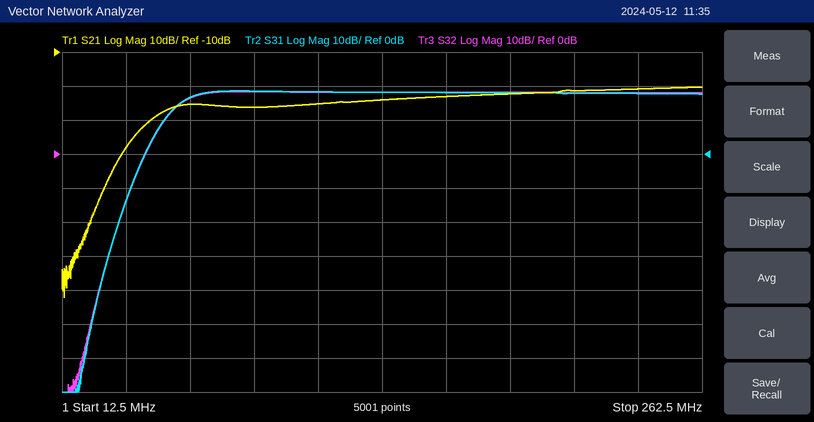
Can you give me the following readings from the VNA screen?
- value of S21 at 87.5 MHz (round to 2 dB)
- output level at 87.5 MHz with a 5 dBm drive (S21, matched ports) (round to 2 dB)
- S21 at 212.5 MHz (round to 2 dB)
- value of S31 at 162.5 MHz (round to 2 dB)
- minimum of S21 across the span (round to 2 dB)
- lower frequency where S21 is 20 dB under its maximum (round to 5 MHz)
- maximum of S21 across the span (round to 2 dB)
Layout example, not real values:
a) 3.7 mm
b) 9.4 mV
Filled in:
a) -26 dB
b) -22 dBm
c) -22 dB
d) 18 dB
e) -82 dB
f) 35 MHz
g) -20 dB
